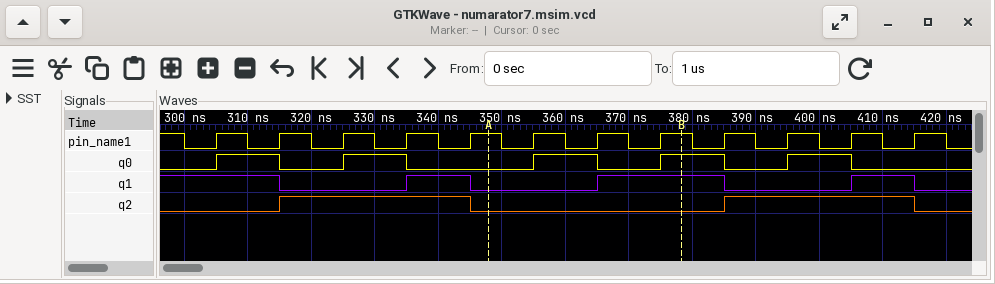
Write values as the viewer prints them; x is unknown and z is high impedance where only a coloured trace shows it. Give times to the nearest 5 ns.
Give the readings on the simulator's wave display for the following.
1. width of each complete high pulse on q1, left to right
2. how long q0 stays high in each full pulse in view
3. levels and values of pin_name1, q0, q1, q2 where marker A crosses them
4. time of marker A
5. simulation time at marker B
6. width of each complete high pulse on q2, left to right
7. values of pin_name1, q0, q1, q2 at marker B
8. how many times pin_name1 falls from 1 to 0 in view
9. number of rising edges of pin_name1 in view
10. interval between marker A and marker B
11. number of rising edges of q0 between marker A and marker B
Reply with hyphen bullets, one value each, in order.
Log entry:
- 10 ns, 20 ns, 10 ns
- 10 ns, 10 ns, 10 ns, 10 ns, 10 ns
- pin_name1=1, q0=0, q1=0, q2=0
- 350 ns
- 380 ns
- 30 ns, 30 ns
- pin_name1=1, q0=1, q1=1, q2=0
- 13
- 12
- 30 ns
- 2
